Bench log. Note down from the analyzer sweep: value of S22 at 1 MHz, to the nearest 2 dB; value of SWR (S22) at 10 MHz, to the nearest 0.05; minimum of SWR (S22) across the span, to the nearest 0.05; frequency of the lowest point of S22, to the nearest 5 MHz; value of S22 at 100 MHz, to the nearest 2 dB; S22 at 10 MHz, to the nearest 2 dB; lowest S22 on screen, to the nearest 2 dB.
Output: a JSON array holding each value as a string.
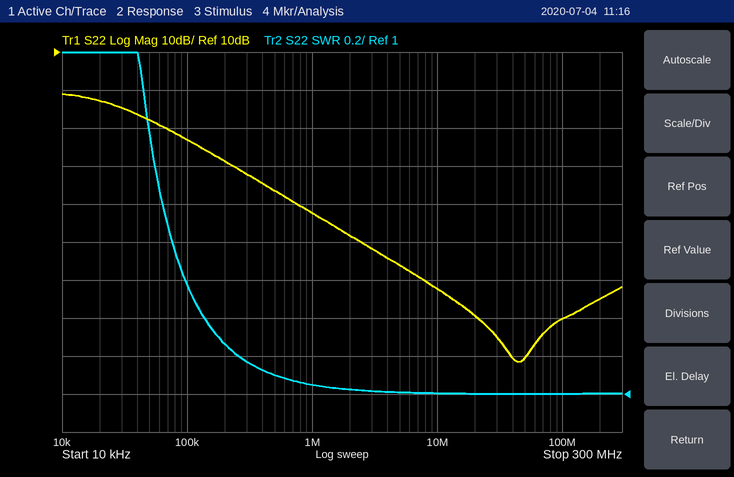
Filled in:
["-32 dB", "1.00", "1.00", "45 MHz", "-60 dB", "-52 dB", "-72 dB"]
